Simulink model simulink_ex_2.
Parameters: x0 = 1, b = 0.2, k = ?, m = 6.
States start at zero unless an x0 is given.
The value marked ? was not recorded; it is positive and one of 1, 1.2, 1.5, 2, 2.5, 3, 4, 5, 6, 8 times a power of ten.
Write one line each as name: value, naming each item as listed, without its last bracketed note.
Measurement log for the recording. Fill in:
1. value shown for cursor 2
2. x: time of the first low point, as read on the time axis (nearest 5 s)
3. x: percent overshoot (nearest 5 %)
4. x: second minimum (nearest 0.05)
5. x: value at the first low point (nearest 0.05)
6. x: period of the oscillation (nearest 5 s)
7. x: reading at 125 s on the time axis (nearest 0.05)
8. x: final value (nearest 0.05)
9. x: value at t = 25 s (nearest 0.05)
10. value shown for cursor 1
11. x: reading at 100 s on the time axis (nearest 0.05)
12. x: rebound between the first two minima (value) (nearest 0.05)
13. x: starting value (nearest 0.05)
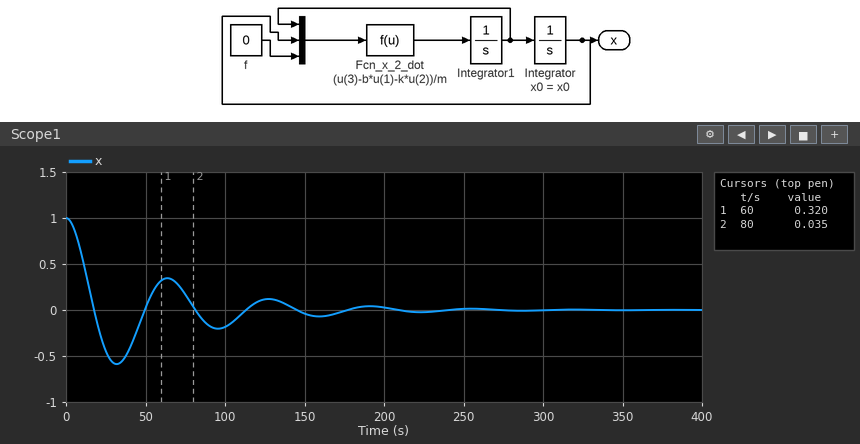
value shown for cursor 2: 0.035
x: time of the first low point, as read on the time axis: 30 s
x: percent overshoot: 60 %
x: second minimum: -0.20
x: value at the first low point: -0.60
x: period of the oscillation: 65 s
x: reading at 125 s on the time axis: 0.10
x: final value: 0.00
x: value at t = 25 s: -0.45
value shown for cursor 1: 0.320
x: reading at 100 s on the time axis: -0.20
x: rebound between the first two minima (value): 0.35
x: starting value: 1.00
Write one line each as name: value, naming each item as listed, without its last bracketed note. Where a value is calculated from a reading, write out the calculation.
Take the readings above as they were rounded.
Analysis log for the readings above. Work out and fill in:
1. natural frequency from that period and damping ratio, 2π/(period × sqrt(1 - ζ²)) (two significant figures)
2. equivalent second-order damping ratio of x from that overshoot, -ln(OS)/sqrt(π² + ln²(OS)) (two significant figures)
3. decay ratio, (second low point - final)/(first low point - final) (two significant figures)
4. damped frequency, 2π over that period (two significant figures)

natural frequency from that period and damping ratio, 2π/(period × sqrt(1 - ζ²)): 2π / (65 × sqrt(1 - 0.16²)) = 0.098 rad/s
equivalent second-order damping ratio of x from that overshoot, -ln(OS)/sqrt(π² + ln²(OS)): ln(0.6) = -0.511; 0.511 / sqrt(9.870 + 0.261) = 0.16
decay ratio, (second low point - final)/(first low point - final): (-0.2 - 0) / (-0.6 - 0) = 0.33
damped frequency, 2π over that period: 2π / 65 = 0.097 rad/s
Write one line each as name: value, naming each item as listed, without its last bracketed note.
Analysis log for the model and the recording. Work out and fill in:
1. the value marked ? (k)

the value marked ?: 0.06
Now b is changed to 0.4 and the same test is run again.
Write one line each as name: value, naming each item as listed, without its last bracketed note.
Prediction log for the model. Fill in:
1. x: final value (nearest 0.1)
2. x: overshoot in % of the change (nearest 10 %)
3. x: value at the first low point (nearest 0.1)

x: final value: 0.0
x: overshoot in % of the change: 30 %
x: value at the first low point: -0.3
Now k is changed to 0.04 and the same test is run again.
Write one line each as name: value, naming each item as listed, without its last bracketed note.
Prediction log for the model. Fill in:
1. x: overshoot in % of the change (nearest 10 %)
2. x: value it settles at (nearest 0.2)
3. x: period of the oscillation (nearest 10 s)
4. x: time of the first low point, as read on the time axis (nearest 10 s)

x: overshoot in % of the change: 50 %
x: value it settles at: 0.0
x: period of the oscillation: 80 s
x: time of the first low point, as read on the time axis: 40 s
